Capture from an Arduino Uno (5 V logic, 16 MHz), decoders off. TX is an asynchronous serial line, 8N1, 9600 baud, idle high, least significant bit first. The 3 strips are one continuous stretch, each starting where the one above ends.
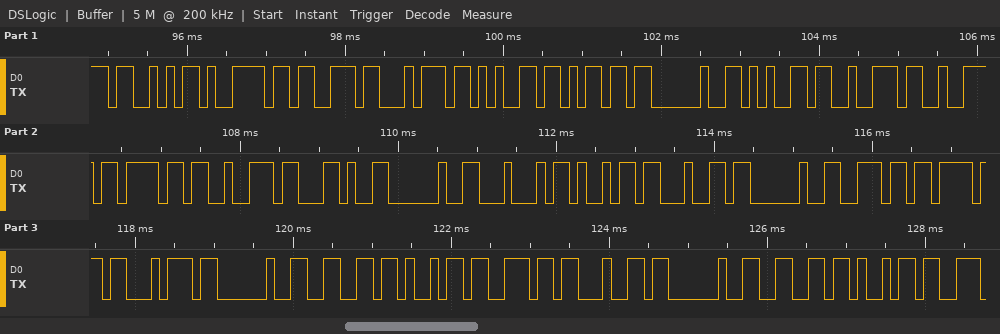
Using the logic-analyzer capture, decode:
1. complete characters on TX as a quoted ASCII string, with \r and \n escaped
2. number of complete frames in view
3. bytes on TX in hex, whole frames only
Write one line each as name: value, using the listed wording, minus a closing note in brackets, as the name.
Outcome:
complete characters on TX as a quoted ASCII string, with \r and \n escaped: "System error, Did not find fi"
number of complete frames in view: 29
bytes on TX in hex, whole frames only: 53 79 73 74 65 6D 20 65 72 72 6F 72 2C 20 44 69 64 20 6E 6F 74 20 66 69 6E 64 20 66 69
